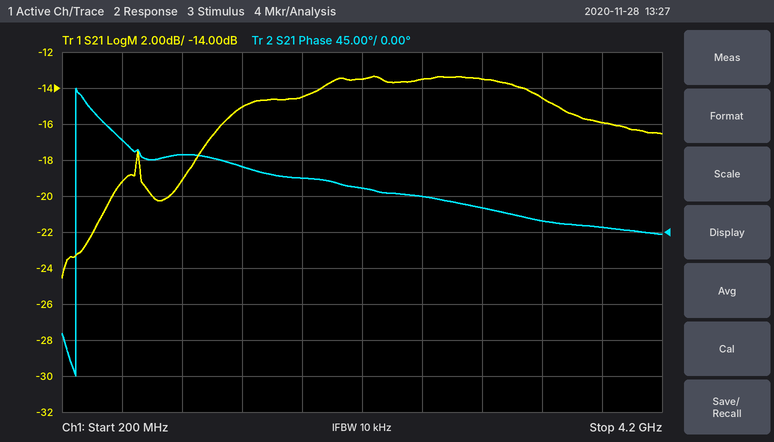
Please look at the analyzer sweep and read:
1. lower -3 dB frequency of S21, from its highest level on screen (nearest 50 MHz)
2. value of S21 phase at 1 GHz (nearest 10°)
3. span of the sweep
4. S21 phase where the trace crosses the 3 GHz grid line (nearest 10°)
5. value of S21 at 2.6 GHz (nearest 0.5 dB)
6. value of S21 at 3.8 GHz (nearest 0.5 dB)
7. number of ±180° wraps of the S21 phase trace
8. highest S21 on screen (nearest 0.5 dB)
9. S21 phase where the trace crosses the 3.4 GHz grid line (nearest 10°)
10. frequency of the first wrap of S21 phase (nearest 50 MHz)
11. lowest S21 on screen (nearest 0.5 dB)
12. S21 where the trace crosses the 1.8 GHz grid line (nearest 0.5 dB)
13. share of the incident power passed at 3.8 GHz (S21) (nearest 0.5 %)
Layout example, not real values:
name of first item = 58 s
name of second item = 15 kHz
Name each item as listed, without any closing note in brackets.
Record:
lower -3 dB frequency of S21, from its highest level on screen = 1.25 GHz
value of S21 phase at 1 GHz = 100°
span of the sweep = 4 GHz
S21 phase where the trace crosses the 3 GHz grid line = 30°
value of S21 at 2.6 GHz = -13.5 dB
value of S21 at 3.8 GHz = -16.0 dB
number of ±180° wraps of the S21 phase trace = 1
highest S21 on screen = -13.5 dB
S21 phase where the trace crosses the 3.4 GHz grid line = 10°
frequency of the first wrap of S21 phase = 300 MHz
lowest S21 on screen = -24.5 dB
S21 where the trace crosses the 1.8 GHz grid line = -14.5 dB
share of the incident power passed at 3.8 GHz (S21) = 2.5 %
